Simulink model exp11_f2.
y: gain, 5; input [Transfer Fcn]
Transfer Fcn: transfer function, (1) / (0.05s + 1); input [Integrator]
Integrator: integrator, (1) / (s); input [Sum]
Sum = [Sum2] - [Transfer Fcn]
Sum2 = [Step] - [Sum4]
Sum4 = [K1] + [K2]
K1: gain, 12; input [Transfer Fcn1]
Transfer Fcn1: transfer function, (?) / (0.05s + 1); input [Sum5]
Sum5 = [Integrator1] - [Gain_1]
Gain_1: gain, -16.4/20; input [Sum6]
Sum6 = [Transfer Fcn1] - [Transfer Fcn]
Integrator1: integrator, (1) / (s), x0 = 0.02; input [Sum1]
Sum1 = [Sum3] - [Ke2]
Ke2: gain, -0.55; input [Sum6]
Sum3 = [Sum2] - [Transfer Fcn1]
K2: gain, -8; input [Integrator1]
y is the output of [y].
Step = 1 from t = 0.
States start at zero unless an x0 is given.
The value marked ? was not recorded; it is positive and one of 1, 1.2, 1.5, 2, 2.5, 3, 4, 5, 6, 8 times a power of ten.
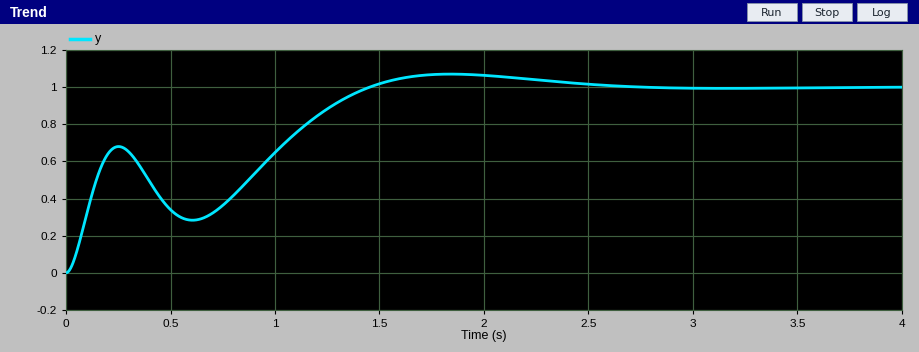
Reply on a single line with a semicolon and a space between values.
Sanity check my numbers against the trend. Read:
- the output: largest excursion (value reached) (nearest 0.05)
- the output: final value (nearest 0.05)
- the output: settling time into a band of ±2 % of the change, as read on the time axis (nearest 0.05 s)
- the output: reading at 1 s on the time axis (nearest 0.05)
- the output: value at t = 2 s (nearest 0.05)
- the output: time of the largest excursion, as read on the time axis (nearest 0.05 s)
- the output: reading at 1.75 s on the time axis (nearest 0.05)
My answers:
1.05; 1.00; 2.45 s; 0.65; 1.05; 1.85 s; 1.05
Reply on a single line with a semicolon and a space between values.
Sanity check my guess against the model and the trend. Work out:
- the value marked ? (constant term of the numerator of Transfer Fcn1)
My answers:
1
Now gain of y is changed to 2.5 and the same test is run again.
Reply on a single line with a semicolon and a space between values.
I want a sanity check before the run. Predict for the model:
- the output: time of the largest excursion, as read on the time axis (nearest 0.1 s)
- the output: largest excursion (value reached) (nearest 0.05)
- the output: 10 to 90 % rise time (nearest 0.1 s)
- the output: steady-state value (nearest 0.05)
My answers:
1.8 s; 0.55; 1.2 s; 0.50
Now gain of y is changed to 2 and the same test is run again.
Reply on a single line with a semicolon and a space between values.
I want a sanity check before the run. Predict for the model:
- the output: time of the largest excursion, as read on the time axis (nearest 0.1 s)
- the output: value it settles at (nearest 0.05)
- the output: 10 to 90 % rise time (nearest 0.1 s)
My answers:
1.8 s; 0.40; 1.2 s
